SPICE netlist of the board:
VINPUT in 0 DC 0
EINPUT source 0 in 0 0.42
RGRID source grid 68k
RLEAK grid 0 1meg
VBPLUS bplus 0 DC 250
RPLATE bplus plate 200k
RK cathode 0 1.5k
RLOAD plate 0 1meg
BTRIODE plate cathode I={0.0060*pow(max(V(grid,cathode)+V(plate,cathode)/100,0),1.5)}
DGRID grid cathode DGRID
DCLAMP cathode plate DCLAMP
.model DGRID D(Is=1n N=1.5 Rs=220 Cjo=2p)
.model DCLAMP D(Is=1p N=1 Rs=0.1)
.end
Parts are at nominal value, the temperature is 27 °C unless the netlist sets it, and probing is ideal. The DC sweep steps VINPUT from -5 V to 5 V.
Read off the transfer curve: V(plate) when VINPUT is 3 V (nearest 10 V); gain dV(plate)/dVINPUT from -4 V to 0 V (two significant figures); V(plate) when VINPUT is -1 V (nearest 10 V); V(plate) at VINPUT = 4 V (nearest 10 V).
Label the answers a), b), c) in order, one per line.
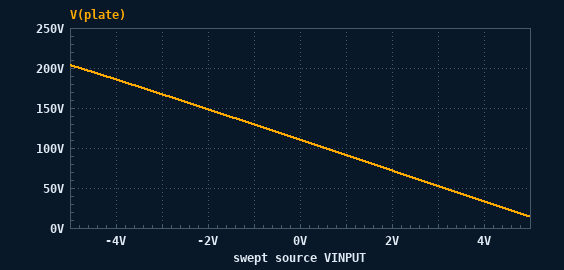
a) 50 V
b) -19 V/V
c) 130 V
d) 30 V
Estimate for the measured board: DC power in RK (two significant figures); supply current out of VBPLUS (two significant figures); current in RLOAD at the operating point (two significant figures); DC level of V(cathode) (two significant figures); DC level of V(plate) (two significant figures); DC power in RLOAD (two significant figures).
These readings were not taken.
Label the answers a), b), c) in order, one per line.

a) 520 µW
b) 700 µA
c) 110 µA
d) 880 mV
e) 110 V
f) 12 mW
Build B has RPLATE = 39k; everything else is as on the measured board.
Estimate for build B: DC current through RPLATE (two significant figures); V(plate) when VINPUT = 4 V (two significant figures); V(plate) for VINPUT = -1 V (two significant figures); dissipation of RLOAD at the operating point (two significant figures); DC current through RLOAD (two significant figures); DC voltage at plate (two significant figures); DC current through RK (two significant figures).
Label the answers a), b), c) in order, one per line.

a) 1.3 mA
b) 170 V
c) 210 V
d) 40 mW
e) 200 µA
f) 200 V
g) 1.1 mA
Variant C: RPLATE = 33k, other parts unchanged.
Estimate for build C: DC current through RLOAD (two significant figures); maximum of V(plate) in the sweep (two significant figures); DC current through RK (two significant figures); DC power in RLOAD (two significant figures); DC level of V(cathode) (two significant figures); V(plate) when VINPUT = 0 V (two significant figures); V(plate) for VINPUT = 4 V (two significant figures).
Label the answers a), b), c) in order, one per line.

a) 210 µA
b) 240 V
c) 1.1 mA
d) 42 mW
e) 1.7 V
f) 210 V
g) 180 V
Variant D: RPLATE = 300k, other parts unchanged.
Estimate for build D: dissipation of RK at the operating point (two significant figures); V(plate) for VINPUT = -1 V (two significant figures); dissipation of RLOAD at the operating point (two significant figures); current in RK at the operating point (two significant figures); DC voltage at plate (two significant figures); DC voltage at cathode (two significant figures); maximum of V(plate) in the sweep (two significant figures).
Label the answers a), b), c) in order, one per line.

a) 310 µW
b) 110 V
c) 7.6 mW
d) 460 µA
e) 87 V
f) 680 mV
g) 190 V
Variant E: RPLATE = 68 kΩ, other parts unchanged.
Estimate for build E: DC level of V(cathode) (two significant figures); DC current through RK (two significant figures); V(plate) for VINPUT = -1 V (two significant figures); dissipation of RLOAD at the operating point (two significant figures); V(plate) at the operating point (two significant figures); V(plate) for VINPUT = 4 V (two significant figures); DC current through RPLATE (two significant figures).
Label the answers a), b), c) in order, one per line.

a) 1.4 V
b) 950 µA
c) 180 V
d) 30 mW
e) 170 V
f) 130 V
g) 1.1 mA
